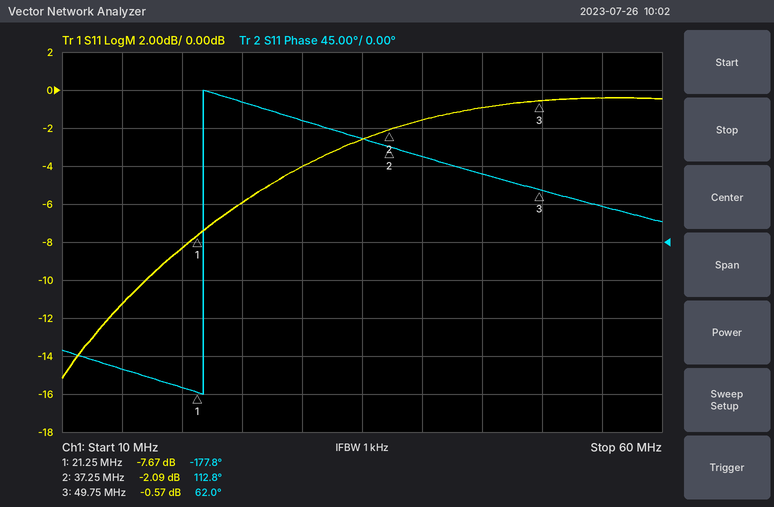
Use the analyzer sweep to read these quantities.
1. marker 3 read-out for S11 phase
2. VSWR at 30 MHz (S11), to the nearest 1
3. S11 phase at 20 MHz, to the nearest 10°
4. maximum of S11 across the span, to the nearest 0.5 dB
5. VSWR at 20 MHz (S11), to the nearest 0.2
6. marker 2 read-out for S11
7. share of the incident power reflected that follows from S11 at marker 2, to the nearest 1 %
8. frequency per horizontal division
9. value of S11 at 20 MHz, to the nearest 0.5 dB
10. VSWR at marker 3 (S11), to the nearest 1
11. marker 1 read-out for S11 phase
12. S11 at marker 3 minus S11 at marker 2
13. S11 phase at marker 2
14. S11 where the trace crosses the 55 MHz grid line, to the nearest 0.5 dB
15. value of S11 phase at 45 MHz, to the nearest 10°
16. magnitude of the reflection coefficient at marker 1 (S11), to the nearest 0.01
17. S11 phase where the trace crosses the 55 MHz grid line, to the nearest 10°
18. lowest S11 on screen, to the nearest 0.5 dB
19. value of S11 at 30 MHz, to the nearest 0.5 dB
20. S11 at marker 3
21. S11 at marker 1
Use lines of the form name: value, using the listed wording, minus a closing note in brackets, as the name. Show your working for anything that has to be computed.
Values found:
marker 3 read-out for S11 phase: 62.0°
VSWR at 30 MHz (S11), to the nearest 1: |Γ| = 10^(-4/20) = 0.6310; VSWR = (1 + 0.6310)/(1 − 0.6310) ≈ 4
S11 phase at 20 MHz, to the nearest 10°: -170°
maximum of S11 across the span, to the nearest 0.5 dB: -0.5 dB
VSWR at 20 MHz (S11), to the nearest 0.2: |Γ| = 10^(-8.5/20) = 0.3758; VSWR = (1 + 0.3758)/(1 − 0.3758) ≈ 2.2
marker 2 read-out for S11: -2.09 dB
share of the incident power reflected that follows from S11 at marker 2, to the nearest 1 %: 10^(-2.09/10) ≈ 62 %
frequency per horizontal division: 5 MHz
value of S11 at 20 MHz, to the nearest 0.5 dB: -8.5 dB
VSWR at marker 3 (S11), to the nearest 1: (1 + 0.9365)/(1 − 0.9365) ≈ 30
marker 1 read-out for S11 phase: -177.8°
S11 at marker 3 minus S11 at marker 2: -0.57 − (-2.09) = 1.52 dB
S11 phase at marker 2: 112.8°
S11 where the trace crosses the 55 MHz grid line, to the nearest 0.5 dB: -0.5 dB
value of S11 phase at 45 MHz, to the nearest 10°: 80°
magnitude of the reflection coefficient at marker 1 (S11), to the nearest 0.01: 10^(-7.67/20) ≈ 0.41
S11 phase where the trace crosses the 55 MHz grid line, to the nearest 10°: 40°
lowest S11 on screen, to the nearest 0.5 dB: -15.0 dB
value of S11 at 30 MHz, to the nearest 0.5 dB: -4.0 dB
S11 at marker 3: -0.57 dB
S11 at marker 1: -7.67 dB
